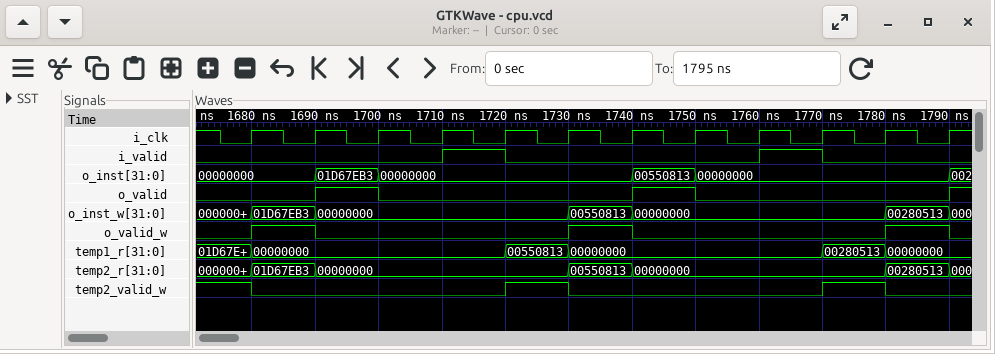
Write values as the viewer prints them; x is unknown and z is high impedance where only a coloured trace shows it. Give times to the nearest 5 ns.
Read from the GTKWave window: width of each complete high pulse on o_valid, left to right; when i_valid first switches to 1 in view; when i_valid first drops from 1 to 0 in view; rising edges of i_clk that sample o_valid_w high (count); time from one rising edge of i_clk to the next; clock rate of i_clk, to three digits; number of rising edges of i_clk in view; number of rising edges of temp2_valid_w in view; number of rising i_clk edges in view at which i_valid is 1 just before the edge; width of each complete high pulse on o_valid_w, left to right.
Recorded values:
10 ns, 10 ns
1710 ns
1720 ns
3
10 ns
100 MHz
12
2
2
10 ns, 10 ns, 10 ns
